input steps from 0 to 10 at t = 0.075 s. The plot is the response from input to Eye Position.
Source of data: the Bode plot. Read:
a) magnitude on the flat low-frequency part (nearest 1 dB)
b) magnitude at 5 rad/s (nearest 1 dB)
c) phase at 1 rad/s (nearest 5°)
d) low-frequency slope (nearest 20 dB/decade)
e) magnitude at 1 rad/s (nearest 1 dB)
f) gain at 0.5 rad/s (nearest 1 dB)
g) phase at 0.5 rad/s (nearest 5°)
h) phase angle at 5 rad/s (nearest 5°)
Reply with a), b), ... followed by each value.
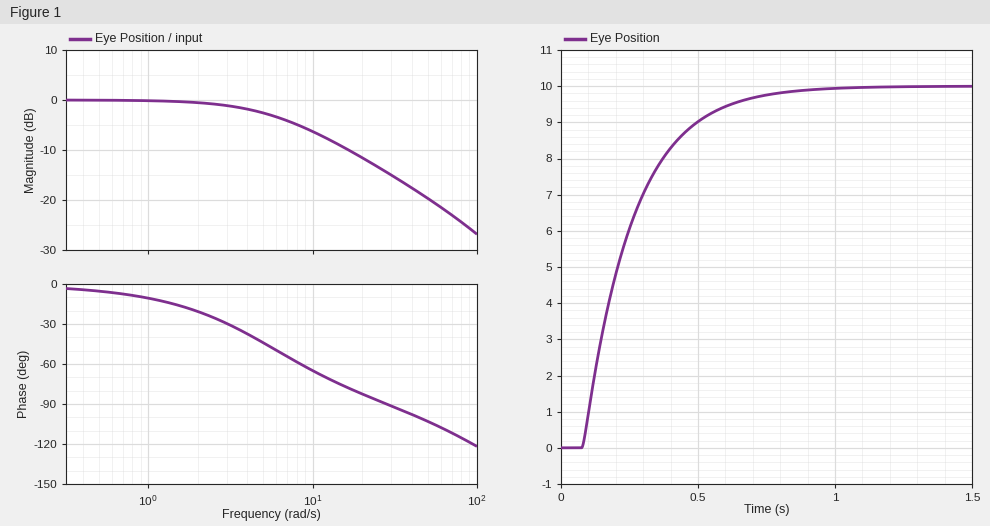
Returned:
a) 0 dB
b) -3 dB
c) -10°
d) 0 dB/decade
e) 0 dB
f) 0 dB
g) -5°
h) -45°
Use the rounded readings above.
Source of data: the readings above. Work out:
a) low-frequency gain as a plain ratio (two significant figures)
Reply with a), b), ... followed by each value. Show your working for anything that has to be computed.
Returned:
a) 10^(0 / 20) = 1.0
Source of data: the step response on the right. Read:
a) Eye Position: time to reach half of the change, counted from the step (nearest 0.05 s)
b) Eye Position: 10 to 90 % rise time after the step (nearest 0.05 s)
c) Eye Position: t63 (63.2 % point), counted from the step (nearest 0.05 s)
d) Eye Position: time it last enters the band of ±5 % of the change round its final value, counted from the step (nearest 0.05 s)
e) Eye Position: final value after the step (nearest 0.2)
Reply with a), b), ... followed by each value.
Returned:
a) 0.15 s
b) 0.40 s
c) 0.20 s
d) 0.55 s
e) 10.0
